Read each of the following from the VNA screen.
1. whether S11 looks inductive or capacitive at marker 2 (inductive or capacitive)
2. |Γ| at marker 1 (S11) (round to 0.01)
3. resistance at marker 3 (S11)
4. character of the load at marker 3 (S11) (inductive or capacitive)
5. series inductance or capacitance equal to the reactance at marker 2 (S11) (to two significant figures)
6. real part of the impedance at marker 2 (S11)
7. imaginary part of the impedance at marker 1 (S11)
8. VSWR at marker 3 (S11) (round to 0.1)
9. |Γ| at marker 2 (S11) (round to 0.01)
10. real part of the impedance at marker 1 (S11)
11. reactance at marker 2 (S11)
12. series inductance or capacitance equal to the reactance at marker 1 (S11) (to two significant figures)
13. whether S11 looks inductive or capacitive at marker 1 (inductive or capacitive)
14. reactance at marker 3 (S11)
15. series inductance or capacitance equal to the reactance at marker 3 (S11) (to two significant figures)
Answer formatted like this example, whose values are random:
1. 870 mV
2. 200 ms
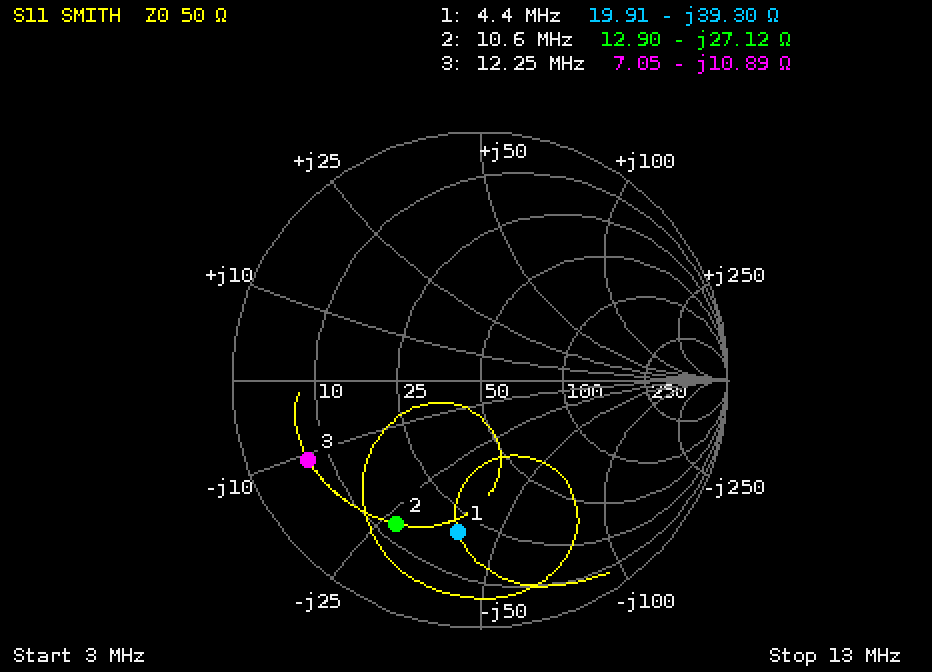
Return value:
1. capacitive
2. 0.62
3. 7.05 Ω
4. capacitive
5. 550 pF
6. 12.90 Ω
7. -39.30 Ω
8. 7.4
9. 0.67
10. 19.91 Ω
11. -27.12 Ω
12. 920 pF
13. capacitive
14. -10.89 Ω
15. 1.2 nF
